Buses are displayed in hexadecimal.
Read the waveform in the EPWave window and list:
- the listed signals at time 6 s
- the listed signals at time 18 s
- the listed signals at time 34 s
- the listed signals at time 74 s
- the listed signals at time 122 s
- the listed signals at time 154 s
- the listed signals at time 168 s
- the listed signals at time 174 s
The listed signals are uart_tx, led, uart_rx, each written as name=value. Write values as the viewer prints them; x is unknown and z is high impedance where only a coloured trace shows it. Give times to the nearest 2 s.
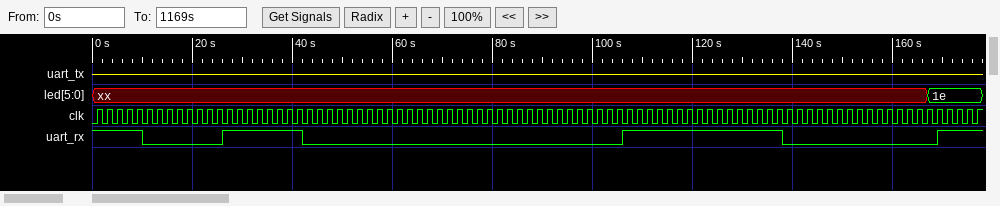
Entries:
uart_tx=z, led=xx, uart_rx=1
uart_tx=z, led=xx, uart_rx=0
uart_tx=z, led=xx, uart_rx=1
uart_tx=z, led=xx, uart_rx=0
uart_tx=z, led=xx, uart_rx=1
uart_tx=z, led=xx, uart_rx=0
uart_tx=z, led=1e, uart_rx=0
uart_tx=z, led=1e, uart_rx=1
